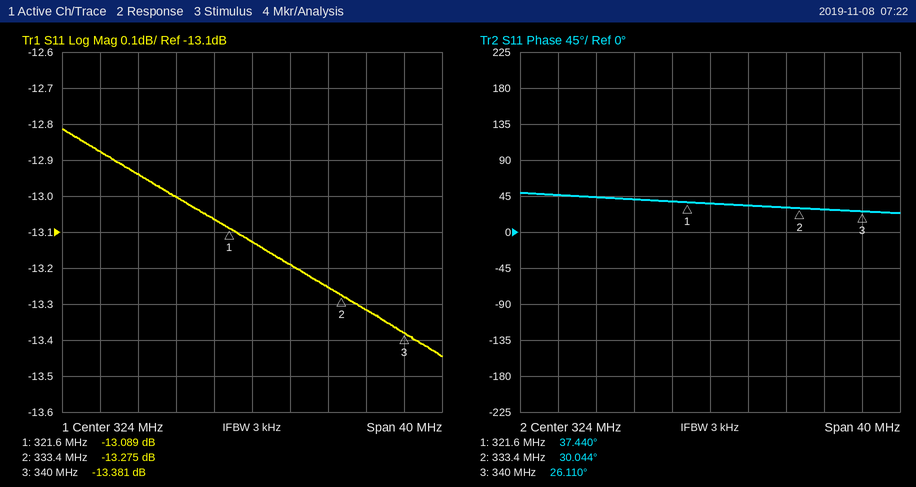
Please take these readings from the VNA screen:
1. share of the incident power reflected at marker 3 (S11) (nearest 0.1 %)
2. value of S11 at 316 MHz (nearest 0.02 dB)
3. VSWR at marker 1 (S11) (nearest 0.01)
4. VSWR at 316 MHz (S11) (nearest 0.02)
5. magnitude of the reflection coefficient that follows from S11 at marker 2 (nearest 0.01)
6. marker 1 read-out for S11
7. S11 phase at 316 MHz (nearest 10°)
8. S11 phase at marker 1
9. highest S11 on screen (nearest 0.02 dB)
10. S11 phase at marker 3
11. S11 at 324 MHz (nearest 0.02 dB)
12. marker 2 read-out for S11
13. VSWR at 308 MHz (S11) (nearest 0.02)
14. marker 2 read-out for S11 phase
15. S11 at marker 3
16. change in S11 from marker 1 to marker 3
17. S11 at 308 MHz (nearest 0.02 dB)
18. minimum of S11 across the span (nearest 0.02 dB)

4.6 %
-13.00 dB
1.57
1.58
0.22
-13.089 dB
40°
37.440°
-12.82 dB
26.110°
-13.12 dB
-13.275 dB
1.58
30.044°
-13.381 dB
-0.292 dB
-12.88 dB
-13.44 dB
